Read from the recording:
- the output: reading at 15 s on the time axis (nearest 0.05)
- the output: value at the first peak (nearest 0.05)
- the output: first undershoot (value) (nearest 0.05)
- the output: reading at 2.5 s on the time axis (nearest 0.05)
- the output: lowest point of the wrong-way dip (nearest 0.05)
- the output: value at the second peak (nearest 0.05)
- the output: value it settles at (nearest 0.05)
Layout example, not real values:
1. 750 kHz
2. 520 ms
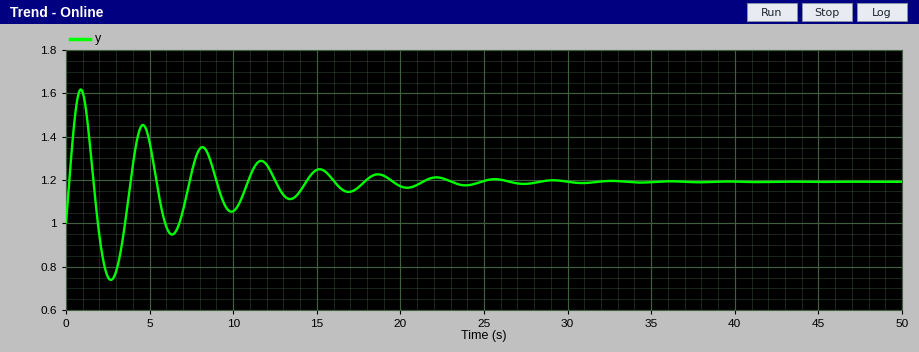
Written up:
1. 1.25
2. 1.60
3. 0.75
4. 0.75
5. 0.75
6. 1.45
7. 1.20
